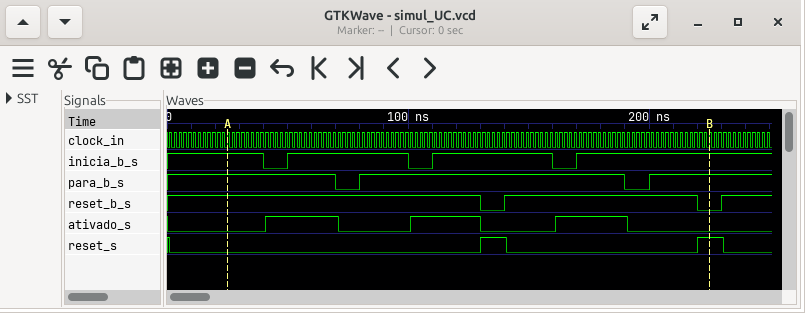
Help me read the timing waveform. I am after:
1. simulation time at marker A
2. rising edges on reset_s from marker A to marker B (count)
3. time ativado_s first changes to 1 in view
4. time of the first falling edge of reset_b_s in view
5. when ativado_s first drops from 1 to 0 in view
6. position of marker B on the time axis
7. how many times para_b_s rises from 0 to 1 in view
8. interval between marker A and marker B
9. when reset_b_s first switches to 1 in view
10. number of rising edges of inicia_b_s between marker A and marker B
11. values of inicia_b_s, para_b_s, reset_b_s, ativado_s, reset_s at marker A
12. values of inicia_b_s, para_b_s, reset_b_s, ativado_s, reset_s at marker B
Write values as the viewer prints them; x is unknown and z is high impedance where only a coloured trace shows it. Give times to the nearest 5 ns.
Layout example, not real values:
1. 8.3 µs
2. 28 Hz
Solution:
1. 25 ns
2. 2
3. 40 ns
4. 130 ns
5. 70 ns
6. 225 ns
7. 2
8. 200 ns
9. 140 ns
10. 3
11. inicia_b_s=1, para_b_s=1, reset_b_s=1, ativado_s=0, reset_s=0
12. inicia_b_s=1, para_b_s=1, reset_b_s=0, ativado_s=0, reset_s=1
